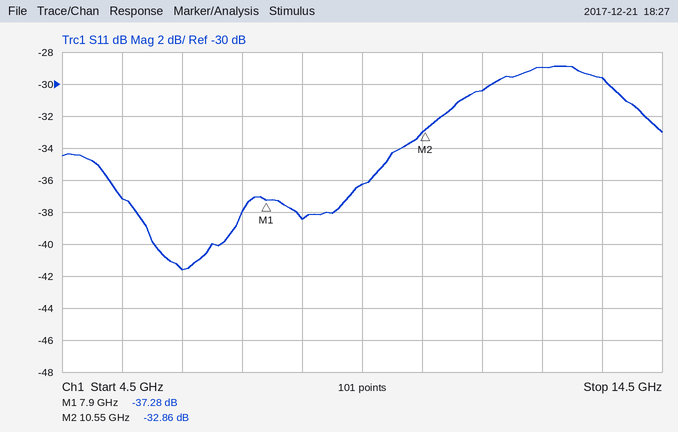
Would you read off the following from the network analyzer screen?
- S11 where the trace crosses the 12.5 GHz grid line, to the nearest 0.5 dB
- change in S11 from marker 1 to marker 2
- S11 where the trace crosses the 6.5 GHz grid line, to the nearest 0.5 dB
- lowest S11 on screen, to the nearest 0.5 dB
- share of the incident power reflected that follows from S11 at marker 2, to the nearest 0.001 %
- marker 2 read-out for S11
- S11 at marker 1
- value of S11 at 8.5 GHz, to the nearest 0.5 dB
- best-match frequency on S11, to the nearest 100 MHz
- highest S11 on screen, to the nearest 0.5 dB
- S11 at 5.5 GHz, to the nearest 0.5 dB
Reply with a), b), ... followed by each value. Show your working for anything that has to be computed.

a) -29.0 dB
b) -32.86 − (-37.28) = 4.42 dB
c) -41.5 dB
d) -41.5 dB
e) 10^(-32.86/10) ≈ 0.052 %
f) -32.86 dB
g) -37.28 dB
h) -38.5 dB
i) 6.5 GHz
j) -29.0 dB
k) -37.0 dB
